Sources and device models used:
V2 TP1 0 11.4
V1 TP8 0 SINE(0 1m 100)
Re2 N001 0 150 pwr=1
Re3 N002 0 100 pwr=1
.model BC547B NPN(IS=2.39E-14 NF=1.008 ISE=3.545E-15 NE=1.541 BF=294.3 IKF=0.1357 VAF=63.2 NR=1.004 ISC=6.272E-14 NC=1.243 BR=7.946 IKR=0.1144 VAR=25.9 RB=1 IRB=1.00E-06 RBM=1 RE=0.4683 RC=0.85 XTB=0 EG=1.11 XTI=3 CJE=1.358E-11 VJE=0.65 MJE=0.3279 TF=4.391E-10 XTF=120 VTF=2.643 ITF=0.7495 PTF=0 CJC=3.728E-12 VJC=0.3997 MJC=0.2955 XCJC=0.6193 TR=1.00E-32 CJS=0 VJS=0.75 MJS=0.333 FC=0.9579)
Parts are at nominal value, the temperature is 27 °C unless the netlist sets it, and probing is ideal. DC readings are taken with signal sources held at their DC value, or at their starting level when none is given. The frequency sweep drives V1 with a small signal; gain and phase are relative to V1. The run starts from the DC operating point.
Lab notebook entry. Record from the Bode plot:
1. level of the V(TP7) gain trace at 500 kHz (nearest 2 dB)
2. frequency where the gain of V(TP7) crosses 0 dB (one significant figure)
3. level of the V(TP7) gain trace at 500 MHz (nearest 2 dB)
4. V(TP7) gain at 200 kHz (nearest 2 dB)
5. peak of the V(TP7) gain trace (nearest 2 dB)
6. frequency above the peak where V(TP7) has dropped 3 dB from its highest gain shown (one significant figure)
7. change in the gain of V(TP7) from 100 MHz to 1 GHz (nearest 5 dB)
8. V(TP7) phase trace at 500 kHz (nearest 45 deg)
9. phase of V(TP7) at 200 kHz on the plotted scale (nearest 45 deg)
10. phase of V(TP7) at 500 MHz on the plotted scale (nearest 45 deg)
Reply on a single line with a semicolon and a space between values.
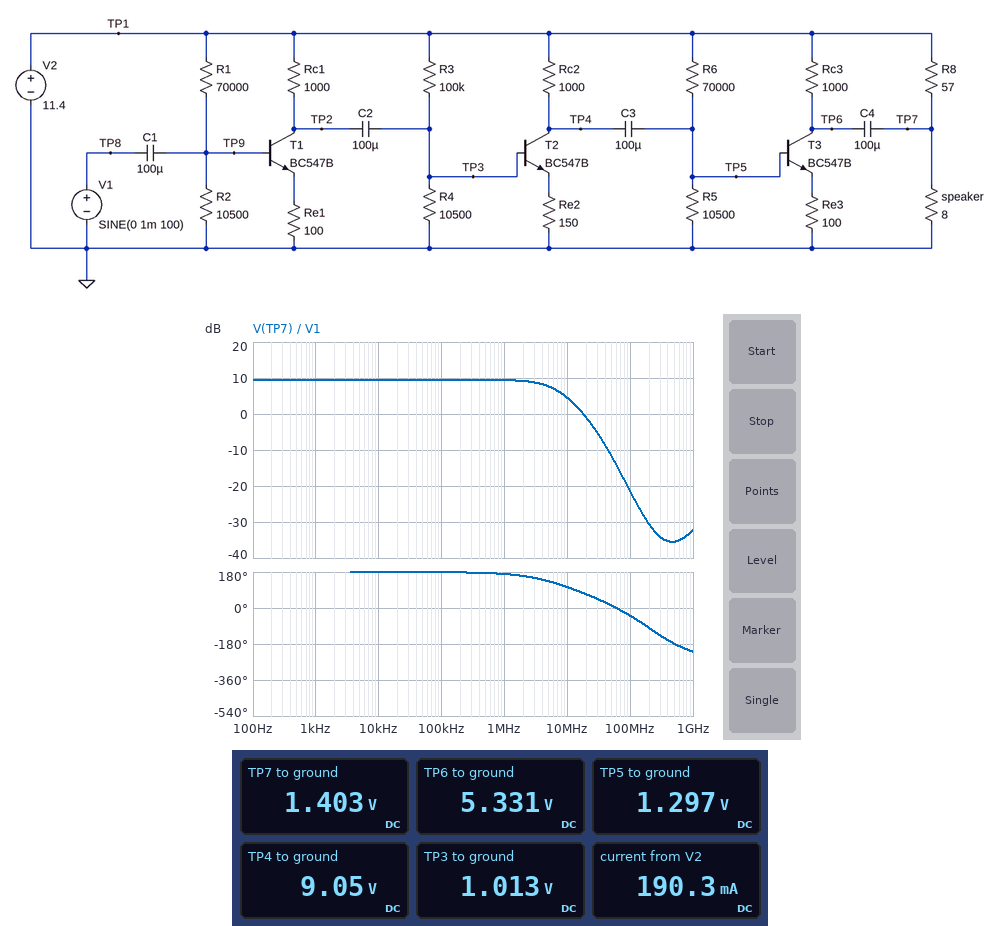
10 dB; 20 MHz; -36 dB; 10 dB; 10 dB; 7 MHz; -10 dB; 180 deg; 180 deg; -180 deg
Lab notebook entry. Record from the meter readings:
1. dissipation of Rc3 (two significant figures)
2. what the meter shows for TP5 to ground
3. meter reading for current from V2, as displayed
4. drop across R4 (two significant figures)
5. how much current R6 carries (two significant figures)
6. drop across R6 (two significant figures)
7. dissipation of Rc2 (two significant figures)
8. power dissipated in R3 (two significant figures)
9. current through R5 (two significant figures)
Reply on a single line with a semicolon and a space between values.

37 mW; 1.297 V; 190.3 mA; 1.0 V; 140 µA; 10 V; 5.5 mW; 1.1 mW; 120 µA
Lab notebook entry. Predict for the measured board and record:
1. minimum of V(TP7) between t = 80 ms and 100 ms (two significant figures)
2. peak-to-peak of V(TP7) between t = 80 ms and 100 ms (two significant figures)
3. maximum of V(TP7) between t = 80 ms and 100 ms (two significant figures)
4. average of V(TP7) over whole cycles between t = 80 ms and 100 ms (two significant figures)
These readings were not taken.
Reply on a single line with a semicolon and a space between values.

1.4 V; 6.0 mV; 1.4 V; 1.4 V
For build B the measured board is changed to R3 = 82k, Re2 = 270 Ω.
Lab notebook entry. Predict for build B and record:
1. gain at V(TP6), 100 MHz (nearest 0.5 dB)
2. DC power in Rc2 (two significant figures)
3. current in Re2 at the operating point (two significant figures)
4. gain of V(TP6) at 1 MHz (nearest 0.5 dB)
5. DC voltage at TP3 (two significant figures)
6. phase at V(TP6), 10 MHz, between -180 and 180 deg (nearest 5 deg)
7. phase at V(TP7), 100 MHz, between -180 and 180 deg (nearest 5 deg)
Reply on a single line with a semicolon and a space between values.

-23.0 dB; 4.5 mW; 2.1 mA; 4.5 dB; 1.2 V; 110 deg; -45 deg
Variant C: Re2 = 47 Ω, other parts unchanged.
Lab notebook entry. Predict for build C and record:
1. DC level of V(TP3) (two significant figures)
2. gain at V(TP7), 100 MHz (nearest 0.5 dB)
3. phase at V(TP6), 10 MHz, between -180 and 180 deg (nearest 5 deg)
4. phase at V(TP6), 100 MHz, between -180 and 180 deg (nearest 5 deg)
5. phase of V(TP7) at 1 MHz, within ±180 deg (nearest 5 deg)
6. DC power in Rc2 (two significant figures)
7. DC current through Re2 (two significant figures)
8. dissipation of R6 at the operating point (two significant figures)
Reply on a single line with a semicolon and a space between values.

920 mV; -18.0 dB; 90 deg; -25 deg; 160 deg; 26 mW; 5.1 mA; 1.5 mW
